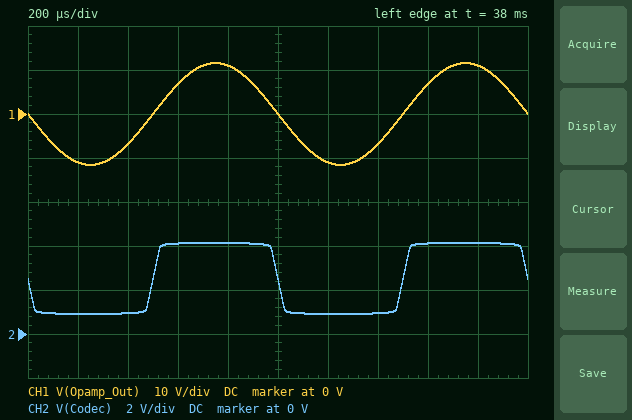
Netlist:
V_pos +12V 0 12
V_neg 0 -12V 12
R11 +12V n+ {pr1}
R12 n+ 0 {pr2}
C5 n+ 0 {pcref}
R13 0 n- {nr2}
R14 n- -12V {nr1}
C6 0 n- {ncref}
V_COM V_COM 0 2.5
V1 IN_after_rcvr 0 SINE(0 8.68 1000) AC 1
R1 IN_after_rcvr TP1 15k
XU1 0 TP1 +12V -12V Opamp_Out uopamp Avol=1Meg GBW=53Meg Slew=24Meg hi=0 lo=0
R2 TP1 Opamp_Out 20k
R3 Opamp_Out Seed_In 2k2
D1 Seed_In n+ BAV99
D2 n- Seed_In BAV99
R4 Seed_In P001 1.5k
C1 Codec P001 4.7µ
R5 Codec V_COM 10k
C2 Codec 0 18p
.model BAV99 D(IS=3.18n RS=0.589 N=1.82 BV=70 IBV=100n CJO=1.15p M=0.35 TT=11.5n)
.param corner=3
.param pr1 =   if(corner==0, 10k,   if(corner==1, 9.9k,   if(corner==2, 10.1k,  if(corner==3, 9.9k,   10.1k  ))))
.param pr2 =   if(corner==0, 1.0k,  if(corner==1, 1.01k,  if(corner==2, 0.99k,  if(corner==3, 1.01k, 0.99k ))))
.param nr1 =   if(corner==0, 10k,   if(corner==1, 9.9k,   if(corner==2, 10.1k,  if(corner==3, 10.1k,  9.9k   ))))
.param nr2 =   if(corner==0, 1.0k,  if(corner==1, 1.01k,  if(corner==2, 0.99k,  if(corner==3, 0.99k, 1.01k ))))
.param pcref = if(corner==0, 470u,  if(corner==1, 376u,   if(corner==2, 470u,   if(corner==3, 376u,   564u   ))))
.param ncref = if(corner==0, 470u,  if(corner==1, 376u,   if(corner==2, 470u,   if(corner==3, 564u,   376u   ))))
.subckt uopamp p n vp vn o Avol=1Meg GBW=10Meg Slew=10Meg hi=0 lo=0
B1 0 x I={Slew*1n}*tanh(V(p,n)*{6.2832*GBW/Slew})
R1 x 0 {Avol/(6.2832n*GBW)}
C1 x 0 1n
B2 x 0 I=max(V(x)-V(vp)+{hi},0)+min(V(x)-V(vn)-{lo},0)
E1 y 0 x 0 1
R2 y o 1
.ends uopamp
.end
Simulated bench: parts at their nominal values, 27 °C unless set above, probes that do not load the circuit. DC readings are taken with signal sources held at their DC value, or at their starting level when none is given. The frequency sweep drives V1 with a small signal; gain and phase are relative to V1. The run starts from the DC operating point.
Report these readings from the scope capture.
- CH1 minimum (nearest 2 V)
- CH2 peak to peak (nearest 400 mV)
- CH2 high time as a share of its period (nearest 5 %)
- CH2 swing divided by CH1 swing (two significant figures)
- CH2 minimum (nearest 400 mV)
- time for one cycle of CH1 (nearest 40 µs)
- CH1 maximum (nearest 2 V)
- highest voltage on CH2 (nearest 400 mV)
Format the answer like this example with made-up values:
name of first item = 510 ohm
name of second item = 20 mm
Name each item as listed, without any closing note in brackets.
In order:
CH1 minimum = -12 V
CH2 peak to peak = 3.2 V
CH2 high time as a share of its period = 50 %
CH2 swing divided by CH1 swing = 0.14
CH2 minimum = 800 mV
time for one cycle of CH1 = 1.00 ms
CH1 maximum = 12 V
highest voltage on CH2 = 4.0 V
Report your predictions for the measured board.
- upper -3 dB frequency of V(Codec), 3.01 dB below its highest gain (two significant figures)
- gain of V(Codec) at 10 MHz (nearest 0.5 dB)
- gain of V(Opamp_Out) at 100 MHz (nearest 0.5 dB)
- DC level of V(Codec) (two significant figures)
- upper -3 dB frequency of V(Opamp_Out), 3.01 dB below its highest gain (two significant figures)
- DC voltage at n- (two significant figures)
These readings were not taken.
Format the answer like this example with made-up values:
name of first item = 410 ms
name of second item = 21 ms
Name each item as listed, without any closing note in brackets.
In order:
upper -3 dB frequency of V(Codec), 3.01 dB below its highest gain = 3.1 MHz
gain of V(Codec) at 10 MHz = -11.5 dB
gain of V(Opamp_Out) at 100 MHz = -10.5 dB
DC level of V(Codec) = 2.5 V
upper -3 dB frequency of V(Opamp_Out), 3.01 dB below its highest gain = 23 MHz
DC voltage at n- = -1.1 V
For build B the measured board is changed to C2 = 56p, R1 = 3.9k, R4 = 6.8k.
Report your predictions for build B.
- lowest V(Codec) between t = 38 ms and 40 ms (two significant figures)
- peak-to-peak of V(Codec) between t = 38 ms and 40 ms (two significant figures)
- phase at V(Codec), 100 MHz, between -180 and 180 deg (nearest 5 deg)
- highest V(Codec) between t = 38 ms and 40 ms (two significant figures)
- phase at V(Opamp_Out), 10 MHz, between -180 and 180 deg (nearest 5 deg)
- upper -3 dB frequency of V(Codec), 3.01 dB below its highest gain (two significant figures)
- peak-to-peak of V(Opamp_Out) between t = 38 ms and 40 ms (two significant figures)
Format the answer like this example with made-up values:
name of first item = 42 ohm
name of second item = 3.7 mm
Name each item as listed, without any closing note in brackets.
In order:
lowest V(Codec) between t = 38 ms and 40 ms = 1.4 V
peak-to-peak of V(Codec) between t = 38 ms and 40 ms = 2.3 V
phase at V(Codec), 100 MHz, between -180 and 180 deg = -55 deg
highest V(Codec) between t = 38 ms and 40 ms = 3.7 V
phase at V(Opamp_Out), 10 MHz, between -180 and 180 deg = 130 deg
upper -3 dB frequency of V(Codec), 3.01 dB below its highest gain = 600 kHz
peak-to-peak of V(Opamp_Out) between t = 38 ms and 40 ms = 24 V
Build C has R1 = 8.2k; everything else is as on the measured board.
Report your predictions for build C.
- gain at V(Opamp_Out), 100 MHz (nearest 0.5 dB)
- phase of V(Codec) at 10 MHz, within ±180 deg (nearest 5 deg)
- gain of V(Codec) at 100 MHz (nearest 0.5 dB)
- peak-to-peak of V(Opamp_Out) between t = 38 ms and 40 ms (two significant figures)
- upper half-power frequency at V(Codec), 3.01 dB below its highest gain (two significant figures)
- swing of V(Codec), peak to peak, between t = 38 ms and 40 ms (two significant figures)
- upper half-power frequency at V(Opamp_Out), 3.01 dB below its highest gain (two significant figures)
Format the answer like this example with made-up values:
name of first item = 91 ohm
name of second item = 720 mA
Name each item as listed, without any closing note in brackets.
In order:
gain at V(Opamp_Out), 100 MHz = -8.5 dB
phase of V(Codec) at 10 MHz, within ±180 deg = 70 deg
gain of V(Codec) at 100 MHz = -44.0 dB
peak-to-peak of V(Opamp_Out) between t = 38 ms and 40 ms = 24 V
upper half-power frequency at V(Codec), 3.01 dB below its highest gain = 3.0 MHz
swing of V(Codec), peak to peak, between t = 38 ms and 40 ms = 3.3 V
upper half-power frequency at V(Opamp_Out), 3.01 dB below its highest gain = 15 MHz
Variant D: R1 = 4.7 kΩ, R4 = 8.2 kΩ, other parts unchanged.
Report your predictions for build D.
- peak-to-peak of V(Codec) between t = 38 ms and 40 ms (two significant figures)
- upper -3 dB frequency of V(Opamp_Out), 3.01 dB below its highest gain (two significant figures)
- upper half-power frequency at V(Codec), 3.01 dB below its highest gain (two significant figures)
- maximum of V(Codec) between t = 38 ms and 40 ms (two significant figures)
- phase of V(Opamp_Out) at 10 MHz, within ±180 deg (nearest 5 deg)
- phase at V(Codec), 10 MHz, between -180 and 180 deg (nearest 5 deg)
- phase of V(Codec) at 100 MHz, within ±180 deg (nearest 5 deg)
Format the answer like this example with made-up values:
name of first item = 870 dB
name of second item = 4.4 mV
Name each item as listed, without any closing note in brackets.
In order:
peak-to-peak of V(Codec) between t = 38 ms and 40 ms = 2.1 V
upper -3 dB frequency of V(Opamp_Out), 3.01 dB below its highest gain = 10 MHz
upper half-power frequency at V(Codec), 3.01 dB below its highest gain = 1.7 MHz
maximum of V(Codec) between t = 38 ms and 40 ms = 3.6 V
phase of V(Opamp_Out) at 10 MHz, within ±180 deg = 135 deg
phase at V(Codec), 10 MHz, between -180 and 180 deg = 45 deg
phase of V(Codec) at 100 MHz, within ±180 deg = -55 deg
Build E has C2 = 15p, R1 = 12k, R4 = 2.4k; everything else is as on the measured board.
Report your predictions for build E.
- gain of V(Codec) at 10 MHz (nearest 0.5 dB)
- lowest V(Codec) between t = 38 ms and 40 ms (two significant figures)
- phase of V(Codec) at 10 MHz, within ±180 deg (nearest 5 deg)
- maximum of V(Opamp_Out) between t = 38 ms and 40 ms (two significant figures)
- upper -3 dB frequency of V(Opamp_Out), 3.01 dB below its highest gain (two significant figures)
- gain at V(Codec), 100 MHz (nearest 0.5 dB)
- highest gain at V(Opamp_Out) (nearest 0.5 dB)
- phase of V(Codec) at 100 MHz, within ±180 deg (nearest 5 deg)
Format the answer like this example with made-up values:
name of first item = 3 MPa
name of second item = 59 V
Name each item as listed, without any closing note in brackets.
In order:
gain of V(Codec) at 10 MHz = -10.0 dB
lowest V(Codec) between t = 38 ms and 40 ms = 1.0 V
phase of V(Codec) at 10 MHz, within ±180 deg = 75 deg
maximum of V(Opamp_Out) between t = 38 ms and 40 ms = 12 V
upper -3 dB frequency of V(Opamp_Out), 3.01 dB below its highest gain = 20 MHz
gain at V(Codec), 100 MHz = -47.0 dB
highest gain at V(Opamp_Out) = 4.5 dB
phase of V(Codec) at 100 MHz, within ±180 deg = -40 deg
